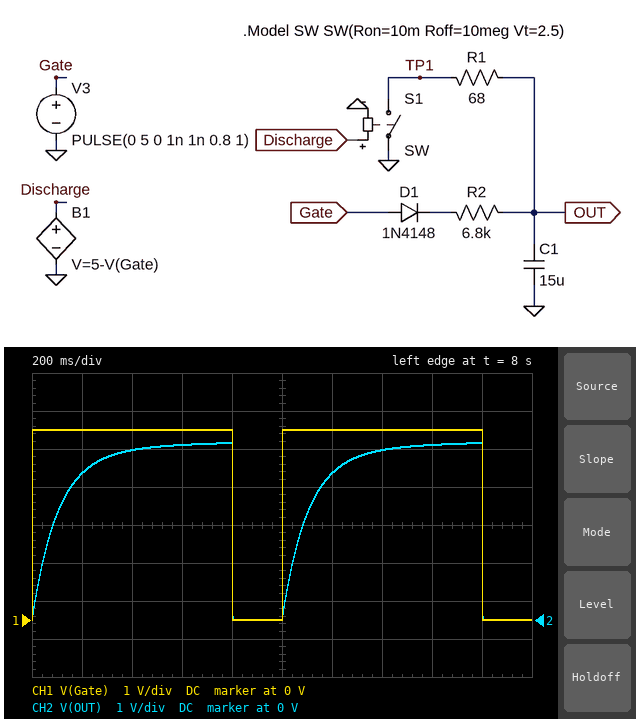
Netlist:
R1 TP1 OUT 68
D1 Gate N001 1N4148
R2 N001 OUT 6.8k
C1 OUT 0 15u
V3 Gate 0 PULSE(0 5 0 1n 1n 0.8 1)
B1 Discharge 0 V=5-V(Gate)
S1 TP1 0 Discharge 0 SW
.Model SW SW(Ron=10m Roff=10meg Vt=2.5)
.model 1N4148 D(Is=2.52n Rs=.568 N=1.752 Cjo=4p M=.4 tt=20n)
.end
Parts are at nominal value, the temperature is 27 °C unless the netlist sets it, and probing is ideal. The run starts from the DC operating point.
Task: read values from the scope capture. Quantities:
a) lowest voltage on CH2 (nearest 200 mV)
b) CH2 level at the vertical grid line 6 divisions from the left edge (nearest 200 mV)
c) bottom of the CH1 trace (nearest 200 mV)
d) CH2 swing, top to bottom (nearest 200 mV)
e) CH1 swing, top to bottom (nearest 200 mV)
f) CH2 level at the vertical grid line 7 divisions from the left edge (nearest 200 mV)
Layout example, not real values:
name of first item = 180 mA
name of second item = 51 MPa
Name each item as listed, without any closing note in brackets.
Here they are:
lowest voltage on CH2 = 0 V
CH2 level at the vertical grid line 6 divisions from the left edge = 3.8 V
bottom of the CH1 trace = 0 V
CH2 swing, top to bottom = 4.6 V
CH1 swing, top to bottom = 5.0 V
CH2 level at the vertical grid line 7 divisions from the left edge = 4.4 V
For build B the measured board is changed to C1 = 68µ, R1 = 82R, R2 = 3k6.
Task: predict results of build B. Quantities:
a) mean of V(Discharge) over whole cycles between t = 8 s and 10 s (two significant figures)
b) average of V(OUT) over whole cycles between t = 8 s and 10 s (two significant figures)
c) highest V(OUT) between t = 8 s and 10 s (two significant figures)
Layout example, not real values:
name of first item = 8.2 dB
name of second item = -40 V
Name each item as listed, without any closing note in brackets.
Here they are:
mean of V(Discharge) over whole cycles between t = 8 s and 10 s = 1.0 V
average of V(OUT) over whole cycles between t = 8 s and 10 s = 2.5 V
highest V(OUT) between t = 8 s and 10 s = 4.3 V
